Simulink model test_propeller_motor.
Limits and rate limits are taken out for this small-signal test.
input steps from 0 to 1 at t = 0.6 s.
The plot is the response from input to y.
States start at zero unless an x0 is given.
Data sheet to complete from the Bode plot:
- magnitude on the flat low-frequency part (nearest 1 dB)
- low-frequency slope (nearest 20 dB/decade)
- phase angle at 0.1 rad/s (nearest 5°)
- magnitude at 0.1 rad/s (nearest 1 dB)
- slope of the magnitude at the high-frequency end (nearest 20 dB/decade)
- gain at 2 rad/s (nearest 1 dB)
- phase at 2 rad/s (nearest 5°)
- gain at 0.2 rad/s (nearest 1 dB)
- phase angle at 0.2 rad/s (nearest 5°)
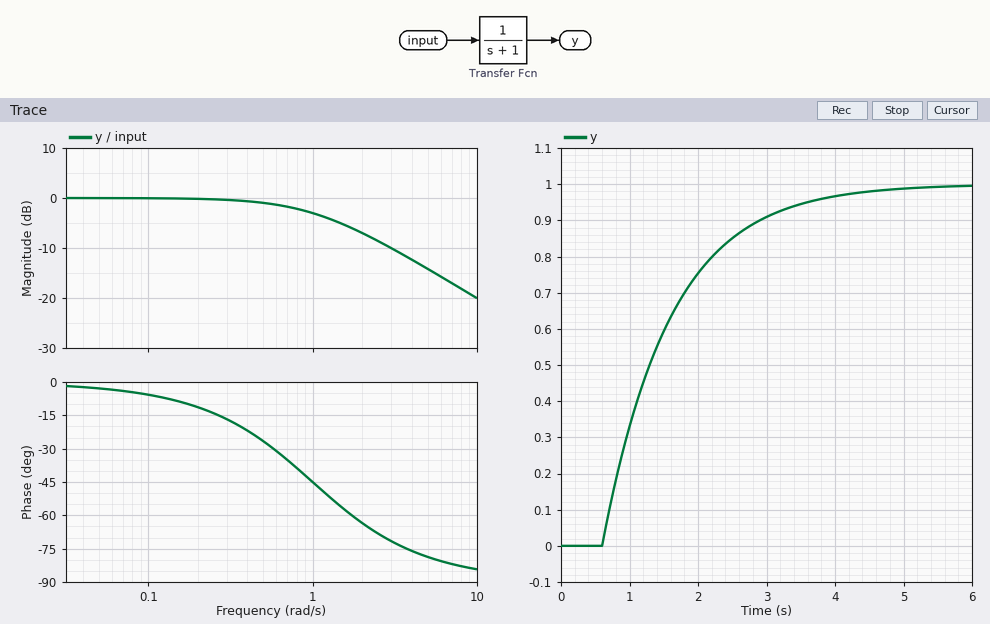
0 dB
0 dB/decade
-5°
0 dB
-20 dB/decade
-7 dB
-65°
0 dB
-10°
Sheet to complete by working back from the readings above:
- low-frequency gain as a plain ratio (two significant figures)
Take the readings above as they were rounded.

1.0
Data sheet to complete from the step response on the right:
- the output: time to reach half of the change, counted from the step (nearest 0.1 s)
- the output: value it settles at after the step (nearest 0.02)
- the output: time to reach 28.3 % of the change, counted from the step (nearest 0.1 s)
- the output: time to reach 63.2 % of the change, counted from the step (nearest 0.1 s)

0.7 s
1.00
0.3 s
1.0 s
